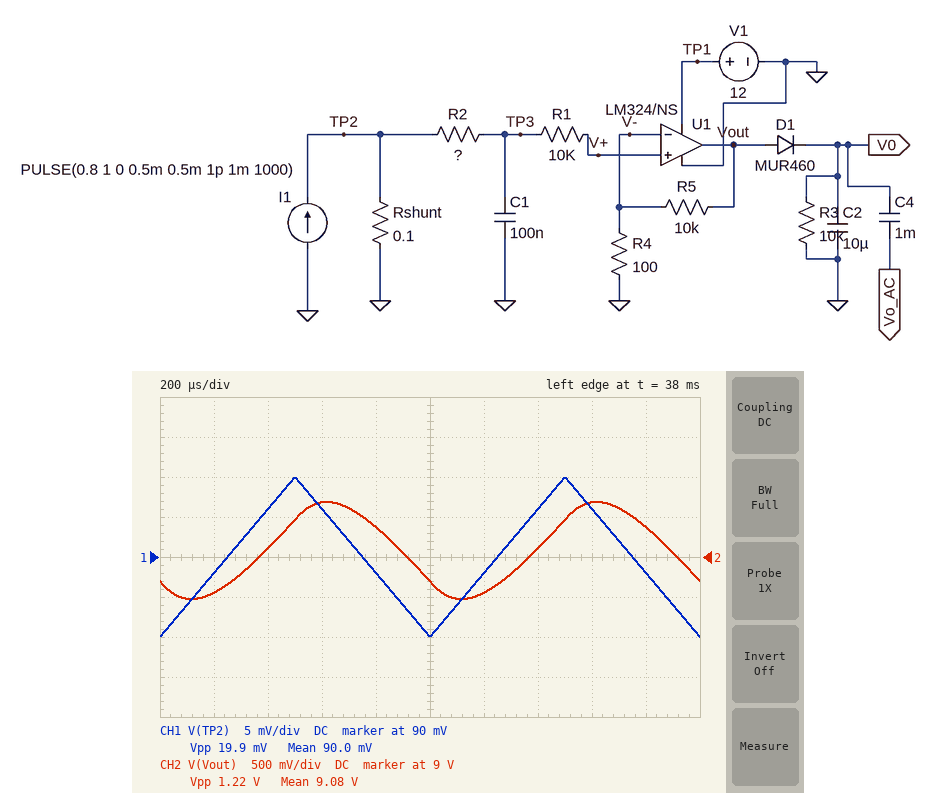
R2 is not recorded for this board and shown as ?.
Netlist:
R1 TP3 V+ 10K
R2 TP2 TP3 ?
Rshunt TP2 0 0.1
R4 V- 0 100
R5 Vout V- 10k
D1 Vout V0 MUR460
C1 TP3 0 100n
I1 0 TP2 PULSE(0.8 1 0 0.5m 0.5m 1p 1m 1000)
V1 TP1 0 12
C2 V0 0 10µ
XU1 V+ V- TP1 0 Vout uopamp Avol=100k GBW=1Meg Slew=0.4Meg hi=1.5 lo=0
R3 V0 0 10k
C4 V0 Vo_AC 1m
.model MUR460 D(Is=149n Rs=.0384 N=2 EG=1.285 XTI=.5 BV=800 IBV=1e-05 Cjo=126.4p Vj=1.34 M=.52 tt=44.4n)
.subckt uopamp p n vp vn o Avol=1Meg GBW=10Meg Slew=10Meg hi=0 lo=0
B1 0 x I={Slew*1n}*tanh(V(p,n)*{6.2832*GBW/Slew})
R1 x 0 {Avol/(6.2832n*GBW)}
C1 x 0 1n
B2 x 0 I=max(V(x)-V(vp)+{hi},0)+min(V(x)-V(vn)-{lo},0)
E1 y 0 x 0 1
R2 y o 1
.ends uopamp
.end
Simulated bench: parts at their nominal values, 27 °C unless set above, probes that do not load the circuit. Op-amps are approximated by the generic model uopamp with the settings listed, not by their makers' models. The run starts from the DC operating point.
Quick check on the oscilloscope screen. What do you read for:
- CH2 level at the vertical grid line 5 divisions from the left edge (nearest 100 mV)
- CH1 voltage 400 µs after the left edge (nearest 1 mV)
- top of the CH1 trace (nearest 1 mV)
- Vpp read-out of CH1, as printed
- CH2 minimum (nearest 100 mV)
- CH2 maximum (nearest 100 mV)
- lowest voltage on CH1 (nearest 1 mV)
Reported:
8.7 V
96 mV
100 mV
19.9 mV
8.5 V
9.7 V
80 mV
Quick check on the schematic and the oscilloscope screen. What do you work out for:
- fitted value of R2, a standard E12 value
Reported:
1.5 kΩ
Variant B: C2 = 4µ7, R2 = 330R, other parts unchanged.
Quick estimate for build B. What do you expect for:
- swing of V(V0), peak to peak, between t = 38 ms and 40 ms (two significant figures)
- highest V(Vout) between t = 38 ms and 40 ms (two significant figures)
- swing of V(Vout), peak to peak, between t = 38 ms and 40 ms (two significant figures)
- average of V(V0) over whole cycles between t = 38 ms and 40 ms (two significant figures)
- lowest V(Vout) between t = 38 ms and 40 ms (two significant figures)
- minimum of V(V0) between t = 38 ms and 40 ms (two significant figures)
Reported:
170 mV
10 V
1.8 V
9.4 V
8.2 V
9.3 V
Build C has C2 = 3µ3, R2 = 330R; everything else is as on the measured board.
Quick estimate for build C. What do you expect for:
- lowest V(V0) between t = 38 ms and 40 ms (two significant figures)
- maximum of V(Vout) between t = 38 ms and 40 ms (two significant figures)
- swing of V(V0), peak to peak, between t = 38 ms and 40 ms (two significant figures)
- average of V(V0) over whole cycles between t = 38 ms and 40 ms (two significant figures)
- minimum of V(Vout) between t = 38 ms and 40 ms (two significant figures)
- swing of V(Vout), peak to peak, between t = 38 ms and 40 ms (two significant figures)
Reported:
9.2 V
10 V
240 mV
9.3 V
8.2 V
1.8 V
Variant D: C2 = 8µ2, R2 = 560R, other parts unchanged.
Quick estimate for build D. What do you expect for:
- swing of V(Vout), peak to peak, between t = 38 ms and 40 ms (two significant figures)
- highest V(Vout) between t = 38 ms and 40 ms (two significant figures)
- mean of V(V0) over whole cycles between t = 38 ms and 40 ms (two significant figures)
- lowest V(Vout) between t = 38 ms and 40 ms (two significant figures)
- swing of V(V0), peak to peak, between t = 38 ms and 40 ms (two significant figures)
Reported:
1.7 V
9.9 V
9.3 V
8.2 V
95 mV
